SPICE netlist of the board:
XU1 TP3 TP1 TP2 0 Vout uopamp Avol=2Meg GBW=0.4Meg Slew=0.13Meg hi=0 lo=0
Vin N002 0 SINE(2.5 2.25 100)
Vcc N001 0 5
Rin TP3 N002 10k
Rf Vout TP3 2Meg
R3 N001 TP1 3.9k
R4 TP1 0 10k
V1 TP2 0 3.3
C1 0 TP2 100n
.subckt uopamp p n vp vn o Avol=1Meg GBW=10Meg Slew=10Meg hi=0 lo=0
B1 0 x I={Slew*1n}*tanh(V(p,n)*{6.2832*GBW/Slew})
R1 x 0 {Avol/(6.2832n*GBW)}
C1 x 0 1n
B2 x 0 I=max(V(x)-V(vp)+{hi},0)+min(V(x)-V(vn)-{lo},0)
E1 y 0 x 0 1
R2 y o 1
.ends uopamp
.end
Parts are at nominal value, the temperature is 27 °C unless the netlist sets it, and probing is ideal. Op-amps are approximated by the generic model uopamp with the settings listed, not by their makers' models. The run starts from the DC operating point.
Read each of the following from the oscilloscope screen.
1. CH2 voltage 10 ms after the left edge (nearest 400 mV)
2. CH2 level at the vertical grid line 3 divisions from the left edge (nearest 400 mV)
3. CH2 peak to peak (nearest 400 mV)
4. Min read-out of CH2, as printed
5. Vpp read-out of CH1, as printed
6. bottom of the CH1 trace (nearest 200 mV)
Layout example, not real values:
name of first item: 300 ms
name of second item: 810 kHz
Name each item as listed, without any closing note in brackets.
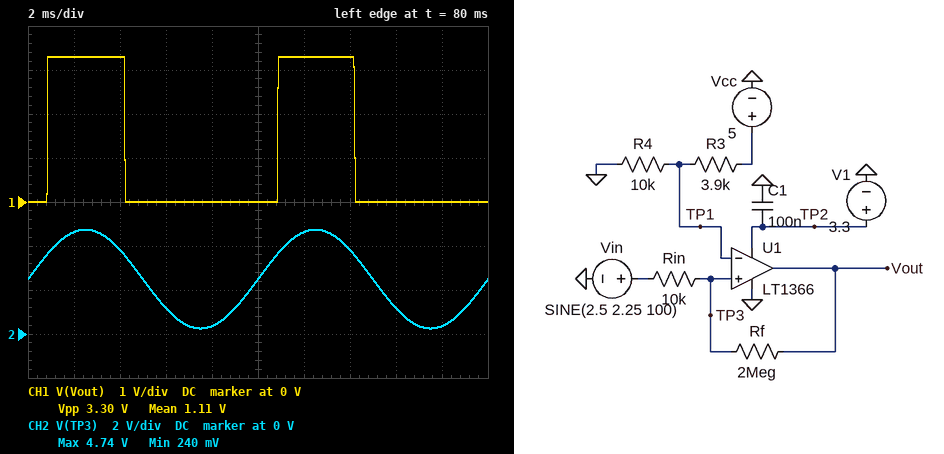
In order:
CH2 voltage 10 ms after the left edge: 2.4 V
CH2 level at the vertical grid line 3 divisions from the left edge: 1.2 V
CH2 peak to peak: 4.4 V
Min read-out of CH2, as printed: 240 mV
Vpp read-out of CH1, as printed: 3.30 V
bottom of the CH1 trace: 0 V
